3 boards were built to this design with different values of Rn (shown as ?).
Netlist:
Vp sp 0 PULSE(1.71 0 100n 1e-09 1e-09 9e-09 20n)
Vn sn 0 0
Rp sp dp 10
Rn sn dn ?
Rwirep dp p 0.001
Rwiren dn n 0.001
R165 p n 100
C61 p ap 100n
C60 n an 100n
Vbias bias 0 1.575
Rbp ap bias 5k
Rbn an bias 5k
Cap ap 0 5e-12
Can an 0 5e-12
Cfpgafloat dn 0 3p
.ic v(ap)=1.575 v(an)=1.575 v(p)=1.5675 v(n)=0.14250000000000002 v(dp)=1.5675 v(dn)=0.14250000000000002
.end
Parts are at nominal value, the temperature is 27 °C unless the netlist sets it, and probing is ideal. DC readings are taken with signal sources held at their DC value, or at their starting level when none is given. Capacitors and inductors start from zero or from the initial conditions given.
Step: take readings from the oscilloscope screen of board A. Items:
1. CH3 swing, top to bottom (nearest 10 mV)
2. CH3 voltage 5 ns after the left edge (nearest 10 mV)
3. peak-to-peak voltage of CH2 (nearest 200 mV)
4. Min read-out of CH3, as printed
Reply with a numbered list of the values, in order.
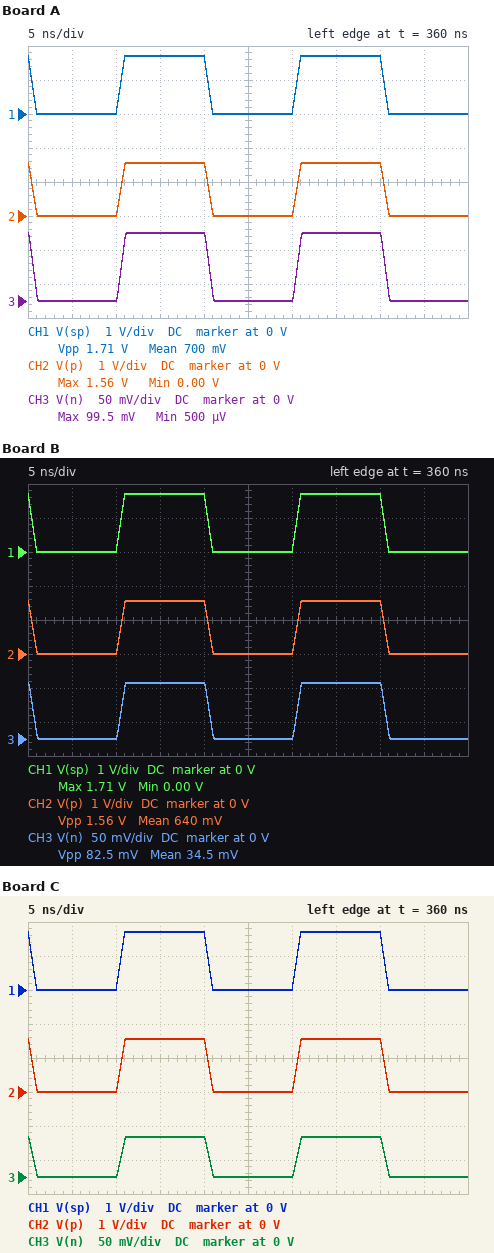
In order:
1. 100 mV
2. 0 V
3. 1.6 V
4. 500 µV
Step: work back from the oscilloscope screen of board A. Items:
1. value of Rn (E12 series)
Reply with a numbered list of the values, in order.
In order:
1. 6.8 Ω
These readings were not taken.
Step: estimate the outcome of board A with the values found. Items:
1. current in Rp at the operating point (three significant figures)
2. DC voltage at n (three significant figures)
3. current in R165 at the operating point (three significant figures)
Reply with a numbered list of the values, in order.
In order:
1. 14.6 mA
2. 99.6 mV
3. 14.6 mA
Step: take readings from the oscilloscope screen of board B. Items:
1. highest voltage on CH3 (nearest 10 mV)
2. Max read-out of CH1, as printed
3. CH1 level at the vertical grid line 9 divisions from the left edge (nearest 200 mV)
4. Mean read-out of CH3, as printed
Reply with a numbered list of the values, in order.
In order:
1. 80 mV
2. 1.71 V
3. 0 V
4. 34.5 mV
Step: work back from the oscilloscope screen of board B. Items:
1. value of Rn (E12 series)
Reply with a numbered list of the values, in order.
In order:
1. 5.6 Ω
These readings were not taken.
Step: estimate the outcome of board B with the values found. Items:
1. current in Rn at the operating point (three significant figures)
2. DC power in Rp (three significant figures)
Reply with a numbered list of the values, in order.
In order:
1. 14.8 mA
2. 2.19 mW
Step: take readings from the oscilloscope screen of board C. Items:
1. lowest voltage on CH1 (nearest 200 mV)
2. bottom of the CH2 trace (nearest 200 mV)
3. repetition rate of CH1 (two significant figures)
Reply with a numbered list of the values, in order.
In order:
1. 0 V
2. 0 V
3. 50 MHz
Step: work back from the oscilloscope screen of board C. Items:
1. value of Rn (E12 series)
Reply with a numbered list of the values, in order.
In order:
1. 3.9 Ω
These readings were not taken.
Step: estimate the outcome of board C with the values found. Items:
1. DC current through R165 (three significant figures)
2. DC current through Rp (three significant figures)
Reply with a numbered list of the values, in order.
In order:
1. 15.0 mA
2. 15.0 mA
